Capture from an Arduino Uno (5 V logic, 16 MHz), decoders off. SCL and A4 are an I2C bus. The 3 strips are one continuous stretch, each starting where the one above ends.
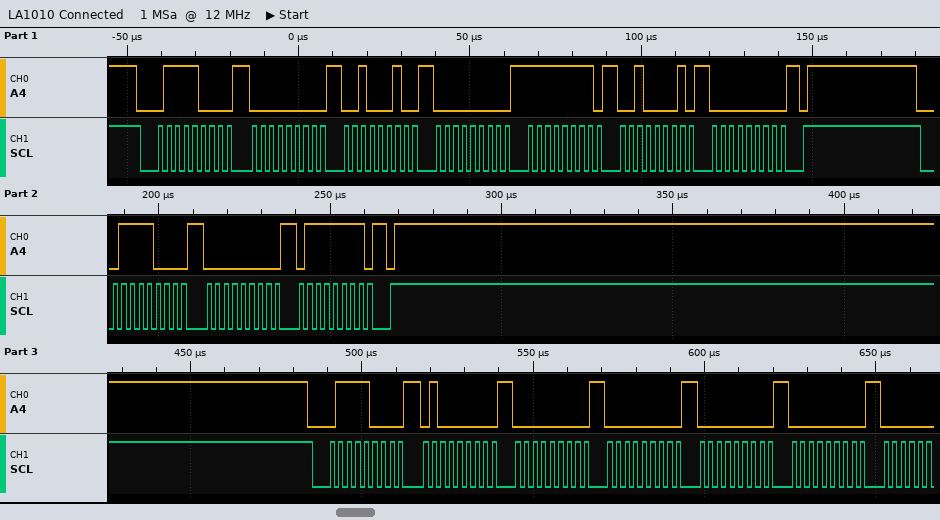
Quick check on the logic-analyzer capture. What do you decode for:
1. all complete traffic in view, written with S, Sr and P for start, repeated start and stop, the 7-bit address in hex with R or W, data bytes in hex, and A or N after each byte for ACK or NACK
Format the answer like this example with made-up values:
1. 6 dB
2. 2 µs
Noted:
1. S 3CW A 00 A 22 A 00 A FF A 21 A 00 A P S 3CW A 00 A 7F A P S 3CW A 40 A 00 A 00 A 00 A 00 A
